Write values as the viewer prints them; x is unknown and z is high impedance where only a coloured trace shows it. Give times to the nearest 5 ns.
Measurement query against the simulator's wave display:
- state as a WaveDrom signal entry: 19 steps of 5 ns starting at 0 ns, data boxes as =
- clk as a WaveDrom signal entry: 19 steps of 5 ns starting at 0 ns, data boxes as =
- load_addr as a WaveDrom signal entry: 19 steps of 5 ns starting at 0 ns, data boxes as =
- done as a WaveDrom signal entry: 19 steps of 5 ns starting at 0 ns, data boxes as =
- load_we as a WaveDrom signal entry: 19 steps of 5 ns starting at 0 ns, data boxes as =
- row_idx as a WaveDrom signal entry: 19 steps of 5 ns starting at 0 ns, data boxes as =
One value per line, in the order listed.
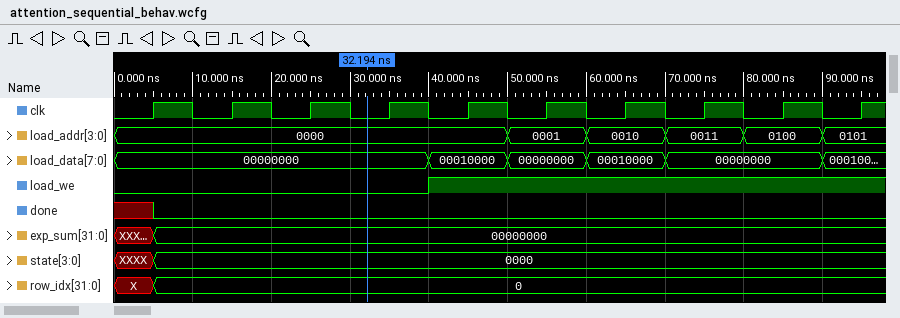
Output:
{name: 'state', wave: 'x=.................', data: '0000'}
{name: 'clk', wave: '0101010101010101010'}
{name: 'load_addr', wave: '=.........=.=.=.=.=', data: '0000 0001 0010 0011 0100 0101'}
{name: 'done', wave: 'x0.................'}
{name: 'load_we', wave: '0.......1..........'}
{name: 'row_idx', wave: 'x=.................', data: '0'}
